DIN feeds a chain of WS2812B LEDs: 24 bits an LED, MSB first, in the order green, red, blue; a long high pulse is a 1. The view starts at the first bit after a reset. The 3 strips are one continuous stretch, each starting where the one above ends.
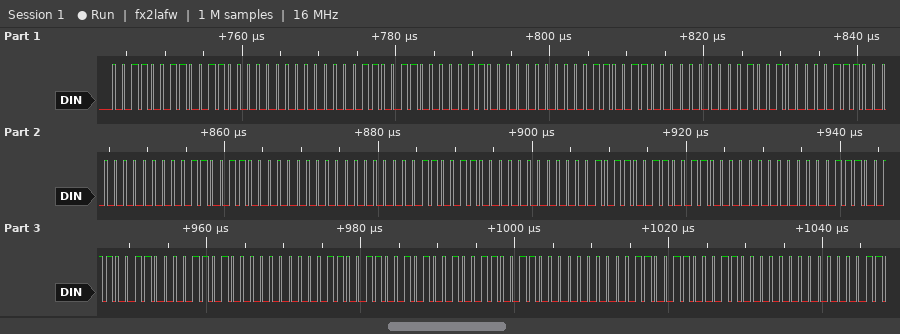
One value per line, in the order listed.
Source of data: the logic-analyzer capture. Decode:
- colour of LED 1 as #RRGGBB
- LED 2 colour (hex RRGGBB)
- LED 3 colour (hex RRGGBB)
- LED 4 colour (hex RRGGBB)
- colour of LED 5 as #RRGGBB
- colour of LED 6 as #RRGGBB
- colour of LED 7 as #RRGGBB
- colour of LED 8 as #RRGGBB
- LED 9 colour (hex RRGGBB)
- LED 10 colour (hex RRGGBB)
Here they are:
#303300
#063300
#003324
#001C33
#000033
#0B0033
#070033
#000D33
#332900
#183300
